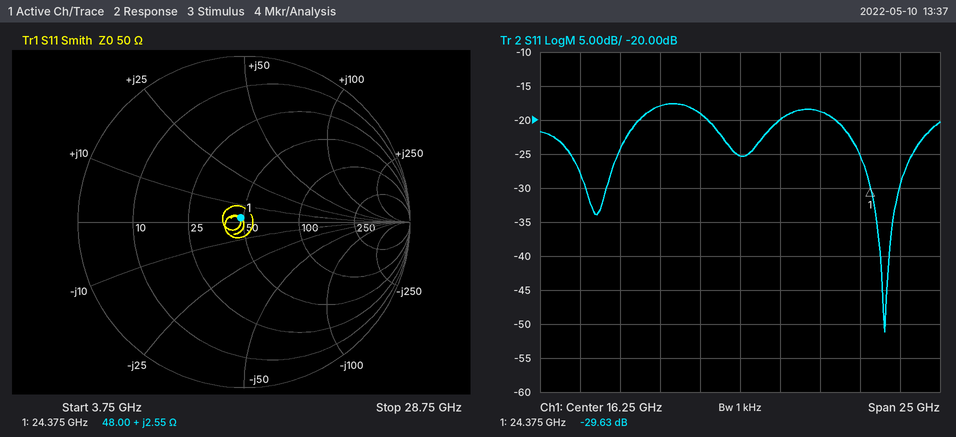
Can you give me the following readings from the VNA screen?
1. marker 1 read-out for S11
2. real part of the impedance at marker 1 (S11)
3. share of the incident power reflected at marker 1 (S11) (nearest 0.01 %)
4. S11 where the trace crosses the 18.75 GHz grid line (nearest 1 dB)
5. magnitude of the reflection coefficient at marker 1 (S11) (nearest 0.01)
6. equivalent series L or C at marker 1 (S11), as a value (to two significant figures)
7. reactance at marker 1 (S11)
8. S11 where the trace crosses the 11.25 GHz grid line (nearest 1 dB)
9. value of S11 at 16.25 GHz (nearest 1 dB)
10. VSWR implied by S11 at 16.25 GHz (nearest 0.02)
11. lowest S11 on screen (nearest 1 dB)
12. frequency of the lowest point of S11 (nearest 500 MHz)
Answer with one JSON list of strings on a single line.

["-29.63 dB", "48.00 Ω", "0.11 %", "-20 dB", "0.03", "17 pH", "+2.55 Ω", "-18 dB", "-25 dB", "1.12", "-51 dB", "25.5 GHz"]
